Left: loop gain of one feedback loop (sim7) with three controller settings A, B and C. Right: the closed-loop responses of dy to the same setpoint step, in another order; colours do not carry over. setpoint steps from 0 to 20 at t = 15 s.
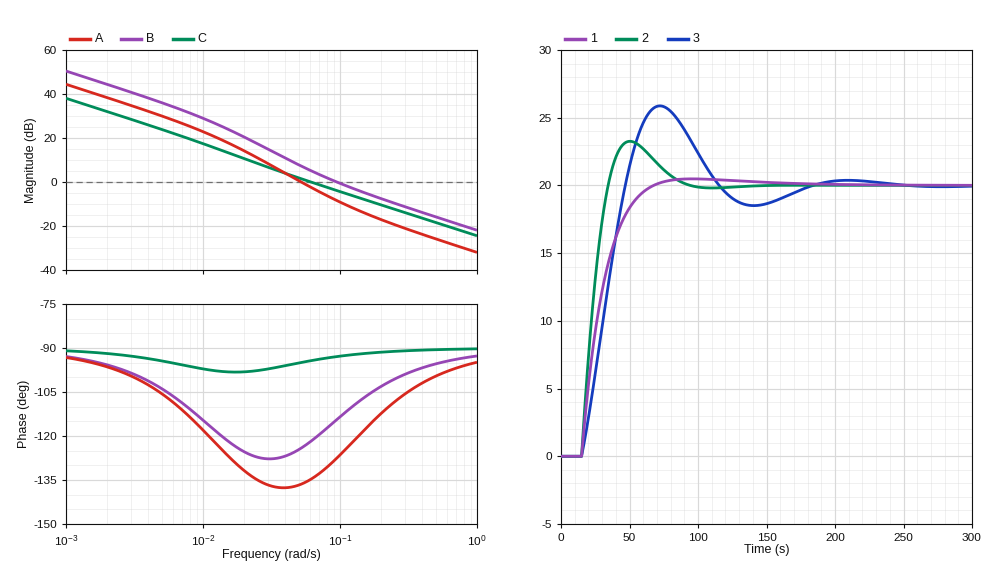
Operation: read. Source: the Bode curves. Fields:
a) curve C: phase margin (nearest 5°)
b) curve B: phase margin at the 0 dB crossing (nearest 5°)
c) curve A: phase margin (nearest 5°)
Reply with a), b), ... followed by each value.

a) 85°
b) 65°
c) 45°
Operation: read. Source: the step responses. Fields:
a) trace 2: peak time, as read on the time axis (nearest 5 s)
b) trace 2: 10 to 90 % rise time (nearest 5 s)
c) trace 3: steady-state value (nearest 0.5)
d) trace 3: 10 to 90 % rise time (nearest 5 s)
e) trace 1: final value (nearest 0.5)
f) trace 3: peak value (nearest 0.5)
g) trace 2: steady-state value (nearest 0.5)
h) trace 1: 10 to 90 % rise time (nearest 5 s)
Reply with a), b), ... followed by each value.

a) 50 s
b) 15 s
c) 20.0
d) 25 s
e) 20.0
f) 26.0
g) 20.0
h) 30 s
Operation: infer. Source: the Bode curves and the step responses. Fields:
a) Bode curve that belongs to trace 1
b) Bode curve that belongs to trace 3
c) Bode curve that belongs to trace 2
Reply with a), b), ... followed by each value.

a) C
b) A
c) B
